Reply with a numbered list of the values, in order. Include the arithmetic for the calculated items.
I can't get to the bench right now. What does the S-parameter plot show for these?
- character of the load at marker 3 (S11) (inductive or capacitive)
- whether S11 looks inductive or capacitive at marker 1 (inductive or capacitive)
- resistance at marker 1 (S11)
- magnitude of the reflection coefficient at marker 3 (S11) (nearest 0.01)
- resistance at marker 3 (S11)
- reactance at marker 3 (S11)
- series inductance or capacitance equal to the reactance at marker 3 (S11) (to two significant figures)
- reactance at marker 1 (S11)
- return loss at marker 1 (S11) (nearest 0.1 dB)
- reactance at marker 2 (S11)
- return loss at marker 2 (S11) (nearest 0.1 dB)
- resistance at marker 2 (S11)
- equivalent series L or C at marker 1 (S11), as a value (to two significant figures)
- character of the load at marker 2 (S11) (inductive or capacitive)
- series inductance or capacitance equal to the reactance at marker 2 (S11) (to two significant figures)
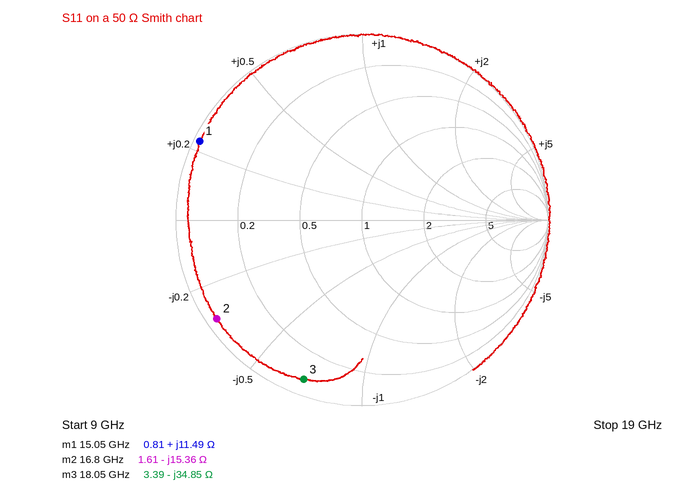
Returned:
1. capacitive
2. inductive
3. 0.81 Ω
4. 0.91
5. 3.39 Ω
6. -34.85 Ω
7. C = 1/(2π × 18.05 GHz × 34.85 Ω) ≈ 253 fF, so 250 fF to two significant figures
8. +11.49 Ω
9. 0.3 dB
10. -15.36 Ω
11. 0.5 dB
12. 1.61 Ω
13. L = 11.49 Ω/(2π × 15.05 GHz) ≈ 122 pH, so 120 pH to two significant figures
14. capacitive
15. C = 1/(2π × 16.8 GHz × 15.36 Ω) ≈ 617 fF, so 620 fF to two significant figures
